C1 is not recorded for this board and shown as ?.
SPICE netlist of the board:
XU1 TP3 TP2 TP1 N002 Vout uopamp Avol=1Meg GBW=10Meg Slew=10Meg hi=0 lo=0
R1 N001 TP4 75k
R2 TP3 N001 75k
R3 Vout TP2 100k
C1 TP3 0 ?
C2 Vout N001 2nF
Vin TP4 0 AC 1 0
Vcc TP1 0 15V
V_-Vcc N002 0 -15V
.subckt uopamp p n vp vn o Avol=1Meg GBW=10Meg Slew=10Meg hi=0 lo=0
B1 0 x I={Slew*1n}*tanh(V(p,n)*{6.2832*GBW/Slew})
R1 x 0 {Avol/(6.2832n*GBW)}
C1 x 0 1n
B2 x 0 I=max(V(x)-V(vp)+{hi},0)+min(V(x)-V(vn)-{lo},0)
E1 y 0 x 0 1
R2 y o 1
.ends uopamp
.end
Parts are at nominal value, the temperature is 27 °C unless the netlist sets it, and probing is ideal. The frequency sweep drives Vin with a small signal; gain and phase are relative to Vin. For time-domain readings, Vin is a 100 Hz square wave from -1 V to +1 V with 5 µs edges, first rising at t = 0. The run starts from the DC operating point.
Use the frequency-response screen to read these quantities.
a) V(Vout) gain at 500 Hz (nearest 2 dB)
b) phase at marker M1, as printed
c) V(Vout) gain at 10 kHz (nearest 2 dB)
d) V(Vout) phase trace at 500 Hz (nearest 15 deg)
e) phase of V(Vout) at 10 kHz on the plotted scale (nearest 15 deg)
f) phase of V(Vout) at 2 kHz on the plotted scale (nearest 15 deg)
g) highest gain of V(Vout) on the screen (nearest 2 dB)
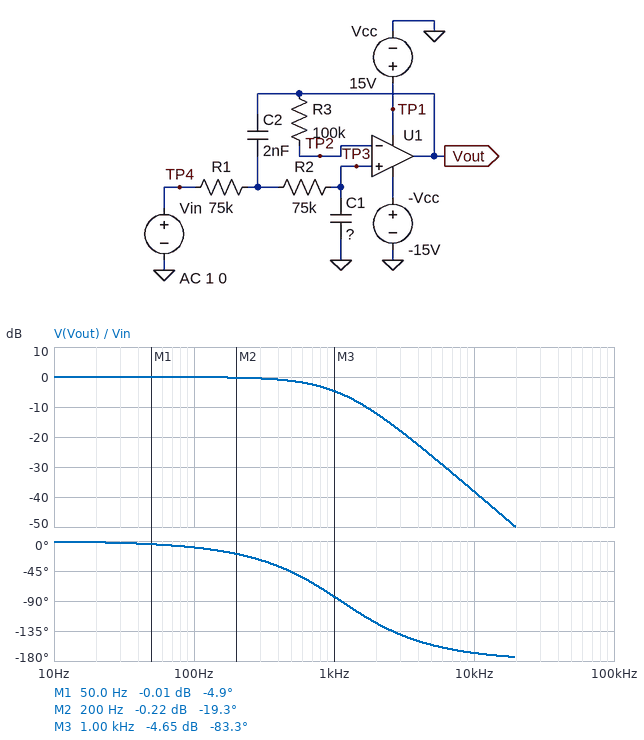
-2 dB
-4.9 deg
-38 dB
-45 deg
-165 deg
-120 deg
0 dB
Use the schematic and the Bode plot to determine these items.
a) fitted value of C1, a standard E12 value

1.8 nF
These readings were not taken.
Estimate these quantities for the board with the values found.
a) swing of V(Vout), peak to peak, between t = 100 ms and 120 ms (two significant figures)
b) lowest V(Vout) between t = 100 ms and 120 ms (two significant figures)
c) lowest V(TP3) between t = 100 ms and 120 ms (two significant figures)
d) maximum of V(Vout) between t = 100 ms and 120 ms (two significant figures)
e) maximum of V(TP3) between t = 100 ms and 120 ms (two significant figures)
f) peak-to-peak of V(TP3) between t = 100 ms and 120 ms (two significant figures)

2.0 V
-1.0 V
-1.0 V
1.0 V
1.0 V
2.0 V
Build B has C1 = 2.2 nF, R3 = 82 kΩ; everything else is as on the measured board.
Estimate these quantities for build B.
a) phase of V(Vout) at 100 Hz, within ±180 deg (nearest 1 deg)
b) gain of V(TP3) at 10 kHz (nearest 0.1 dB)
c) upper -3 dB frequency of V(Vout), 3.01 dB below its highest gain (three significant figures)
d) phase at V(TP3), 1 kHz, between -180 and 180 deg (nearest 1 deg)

-12 deg
-39.9 dB
609 Hz
-89 deg
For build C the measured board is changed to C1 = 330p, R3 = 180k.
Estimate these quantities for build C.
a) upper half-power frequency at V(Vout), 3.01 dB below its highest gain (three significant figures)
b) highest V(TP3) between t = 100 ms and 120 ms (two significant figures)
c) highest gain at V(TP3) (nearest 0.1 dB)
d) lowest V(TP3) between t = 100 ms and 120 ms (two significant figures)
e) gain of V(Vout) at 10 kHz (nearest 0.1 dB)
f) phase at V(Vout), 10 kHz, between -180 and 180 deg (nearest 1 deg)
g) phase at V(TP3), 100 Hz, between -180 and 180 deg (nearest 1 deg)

3.10 kHz
1.5 V
2.6 dB
-1.5 V
-22.9 dB
-167 deg
-2 deg
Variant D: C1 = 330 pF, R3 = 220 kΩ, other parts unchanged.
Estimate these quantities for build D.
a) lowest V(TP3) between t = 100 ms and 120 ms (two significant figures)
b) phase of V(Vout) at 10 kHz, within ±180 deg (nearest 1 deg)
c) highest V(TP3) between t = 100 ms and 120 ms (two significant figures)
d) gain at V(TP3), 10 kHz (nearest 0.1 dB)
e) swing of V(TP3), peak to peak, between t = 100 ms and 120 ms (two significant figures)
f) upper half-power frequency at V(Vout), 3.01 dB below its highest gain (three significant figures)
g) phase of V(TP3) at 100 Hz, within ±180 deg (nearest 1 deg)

-1.5 V
-167 deg
1.5 V
-22.9 dB
3.0 V
3.10 kHz
-2 deg
